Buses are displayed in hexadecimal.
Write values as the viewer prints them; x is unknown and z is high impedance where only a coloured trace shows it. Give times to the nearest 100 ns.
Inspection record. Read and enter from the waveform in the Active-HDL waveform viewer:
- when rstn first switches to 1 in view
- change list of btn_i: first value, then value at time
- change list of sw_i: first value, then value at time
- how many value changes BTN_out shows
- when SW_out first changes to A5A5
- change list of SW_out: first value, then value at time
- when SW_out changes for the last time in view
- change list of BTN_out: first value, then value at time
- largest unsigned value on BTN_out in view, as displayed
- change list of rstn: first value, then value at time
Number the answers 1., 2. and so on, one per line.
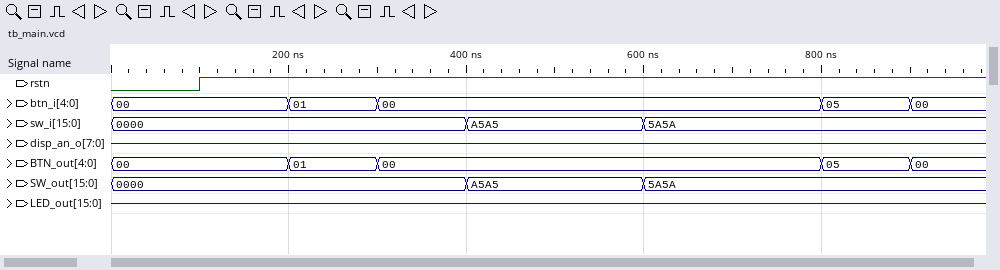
1. 100 ns
2. 00, 01 at 200 ns, 00 at 300 ns, 05 at 800 ns, 00 at 900 ns
3. 0000, A5A5 at 400 ns, 5A5A at 600 ns
4. 4
5. 400 ns
6. 0000, A5A5 at 400 ns, 5A5A at 600 ns
7. 600 ns
8. 00, 01 at 200 ns, 00 at 300 ns, 05 at 800 ns, 00 at 900 ns
9. 05
10. 0, 1 at 100 ns
